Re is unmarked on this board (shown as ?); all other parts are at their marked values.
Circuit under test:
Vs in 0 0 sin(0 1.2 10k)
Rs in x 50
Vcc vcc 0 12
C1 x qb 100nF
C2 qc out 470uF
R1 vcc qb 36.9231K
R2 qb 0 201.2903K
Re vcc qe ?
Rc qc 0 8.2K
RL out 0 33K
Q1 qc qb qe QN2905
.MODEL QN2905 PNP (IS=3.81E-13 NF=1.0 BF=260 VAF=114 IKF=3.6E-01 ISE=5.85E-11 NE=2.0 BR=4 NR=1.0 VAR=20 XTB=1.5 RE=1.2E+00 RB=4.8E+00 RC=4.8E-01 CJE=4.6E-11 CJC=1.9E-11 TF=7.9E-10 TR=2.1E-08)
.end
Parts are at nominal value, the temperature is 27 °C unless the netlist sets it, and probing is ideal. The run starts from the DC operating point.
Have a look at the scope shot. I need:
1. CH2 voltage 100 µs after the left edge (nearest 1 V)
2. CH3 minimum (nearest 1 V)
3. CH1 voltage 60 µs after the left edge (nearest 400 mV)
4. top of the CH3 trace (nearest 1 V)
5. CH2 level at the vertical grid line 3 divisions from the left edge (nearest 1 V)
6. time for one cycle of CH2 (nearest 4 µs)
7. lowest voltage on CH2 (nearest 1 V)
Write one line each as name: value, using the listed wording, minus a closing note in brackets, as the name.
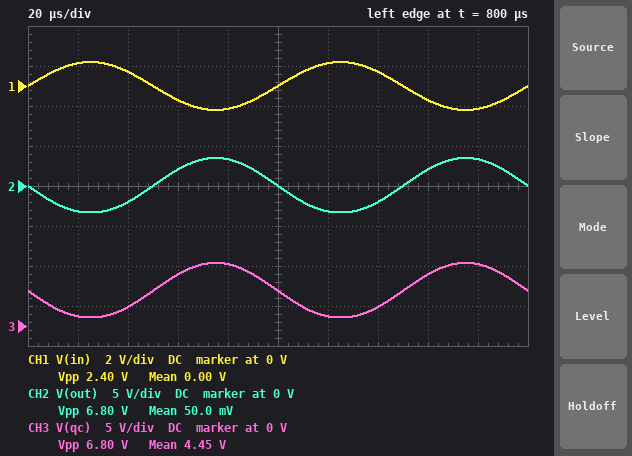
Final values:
CH2 voltage 100 µs after the left edge: 0 V
CH3 minimum: 1 V
CH1 voltage 60 µs after the left edge: -800 mV
top of the CH3 trace: 8 V
CH2 level at the vertical grid line 3 divisions from the left edge: 2 V
time for one cycle of CH2: 100 µs
lowest voltage on CH2: -3 V
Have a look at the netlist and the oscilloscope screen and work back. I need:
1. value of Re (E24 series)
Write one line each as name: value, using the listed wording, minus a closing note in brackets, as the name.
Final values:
value of Re: 2.2 kΩ
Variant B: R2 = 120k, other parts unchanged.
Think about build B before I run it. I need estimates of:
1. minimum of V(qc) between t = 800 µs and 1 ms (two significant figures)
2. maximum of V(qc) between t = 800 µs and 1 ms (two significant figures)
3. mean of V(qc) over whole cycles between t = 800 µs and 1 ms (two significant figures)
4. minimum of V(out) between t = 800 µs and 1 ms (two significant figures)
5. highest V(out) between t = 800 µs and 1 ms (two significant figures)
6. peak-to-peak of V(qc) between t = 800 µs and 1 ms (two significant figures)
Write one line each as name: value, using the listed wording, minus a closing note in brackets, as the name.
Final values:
minimum of V(qc) between t = 800 µs and 1 ms: 3.3 V
maximum of V(qc) between t = 800 µs and 1 ms: 9.3 V
mean of V(qc) over whole cycles between t = 800 µs and 1 ms: 6.6 V
minimum of V(out) between t = 800 µs and 1 ms: -4.4 V
highest V(out) between t = 800 µs and 1 ms: 1.6 V
peak-to-peak of V(qc) between t = 800 µs and 1 ms: 6.0 V
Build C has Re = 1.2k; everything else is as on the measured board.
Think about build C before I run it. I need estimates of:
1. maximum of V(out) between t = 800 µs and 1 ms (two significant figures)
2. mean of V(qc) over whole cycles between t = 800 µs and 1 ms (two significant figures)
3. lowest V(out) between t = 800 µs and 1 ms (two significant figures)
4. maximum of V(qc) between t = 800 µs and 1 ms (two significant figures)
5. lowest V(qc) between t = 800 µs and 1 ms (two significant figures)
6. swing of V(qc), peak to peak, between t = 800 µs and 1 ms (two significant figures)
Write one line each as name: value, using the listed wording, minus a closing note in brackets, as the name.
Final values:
maximum of V(out) between t = 800 µs and 1 ms: 2.8 V
mean of V(qc) over whole cycles between t = 800 µs and 1 ms: 5.6 V
lowest V(out) between t = 800 µs and 1 ms: -6.0 V
maximum of V(qc) between t = 800 µs and 1 ms: 10 V
lowest V(qc) between t = 800 µs and 1 ms: 1.5 V
swing of V(qc), peak to peak, between t = 800 µs and 1 ms: 8.8 V
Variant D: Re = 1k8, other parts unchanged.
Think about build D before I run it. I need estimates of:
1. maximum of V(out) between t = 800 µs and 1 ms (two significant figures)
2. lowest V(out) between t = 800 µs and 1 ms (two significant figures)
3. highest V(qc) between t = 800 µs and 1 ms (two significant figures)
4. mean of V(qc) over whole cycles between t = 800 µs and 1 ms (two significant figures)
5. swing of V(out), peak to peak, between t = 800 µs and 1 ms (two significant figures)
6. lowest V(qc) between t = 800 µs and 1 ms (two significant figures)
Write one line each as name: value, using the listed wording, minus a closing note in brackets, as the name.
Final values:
maximum of V(out) between t = 800 µs and 1 ms: 4.3 V
lowest V(out) between t = 800 µs and 1 ms: -4.0 V
highest V(qc) between t = 800 µs and 1 ms: 9.5 V
mean of V(qc) over whole cycles between t = 800 µs and 1 ms: 5.3 V
swing of V(out), peak to peak, between t = 800 µs and 1 ms: 8.3 V
lowest V(qc) between t = 800 µs and 1 ms: 1.2 V
